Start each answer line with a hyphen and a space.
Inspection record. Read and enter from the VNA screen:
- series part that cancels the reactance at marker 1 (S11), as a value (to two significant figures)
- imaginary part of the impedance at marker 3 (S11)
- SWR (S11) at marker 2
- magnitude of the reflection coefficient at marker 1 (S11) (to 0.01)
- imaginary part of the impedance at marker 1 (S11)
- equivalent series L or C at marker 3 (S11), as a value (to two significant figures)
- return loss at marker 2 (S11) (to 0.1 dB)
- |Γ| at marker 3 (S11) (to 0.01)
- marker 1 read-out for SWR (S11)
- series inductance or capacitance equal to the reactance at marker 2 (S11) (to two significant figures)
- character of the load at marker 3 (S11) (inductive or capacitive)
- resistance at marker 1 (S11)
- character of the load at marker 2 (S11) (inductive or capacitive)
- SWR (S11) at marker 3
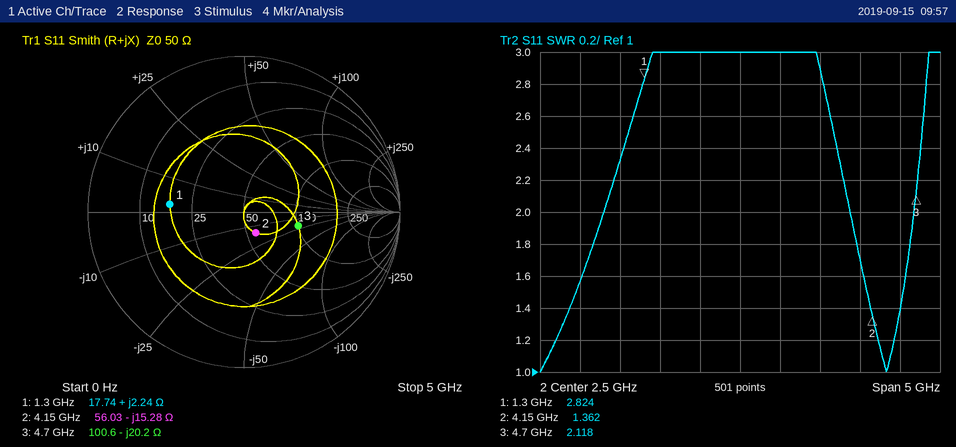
- 55 pF
- -20.2 Ω
- 1.362
- 0.48
- +2.24 Ω
- 1.7 pF
- 16.3 dB
- 0.36
- 2.824
- 2.5 pF
- capacitive
- 17.74 Ω
- capacitive
- 2.118
